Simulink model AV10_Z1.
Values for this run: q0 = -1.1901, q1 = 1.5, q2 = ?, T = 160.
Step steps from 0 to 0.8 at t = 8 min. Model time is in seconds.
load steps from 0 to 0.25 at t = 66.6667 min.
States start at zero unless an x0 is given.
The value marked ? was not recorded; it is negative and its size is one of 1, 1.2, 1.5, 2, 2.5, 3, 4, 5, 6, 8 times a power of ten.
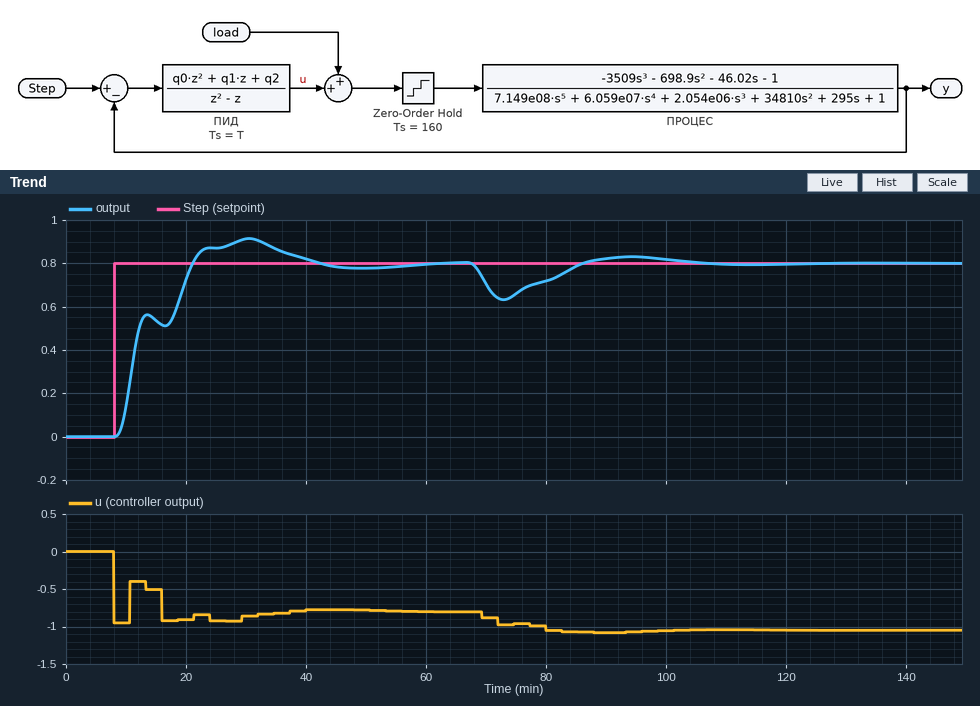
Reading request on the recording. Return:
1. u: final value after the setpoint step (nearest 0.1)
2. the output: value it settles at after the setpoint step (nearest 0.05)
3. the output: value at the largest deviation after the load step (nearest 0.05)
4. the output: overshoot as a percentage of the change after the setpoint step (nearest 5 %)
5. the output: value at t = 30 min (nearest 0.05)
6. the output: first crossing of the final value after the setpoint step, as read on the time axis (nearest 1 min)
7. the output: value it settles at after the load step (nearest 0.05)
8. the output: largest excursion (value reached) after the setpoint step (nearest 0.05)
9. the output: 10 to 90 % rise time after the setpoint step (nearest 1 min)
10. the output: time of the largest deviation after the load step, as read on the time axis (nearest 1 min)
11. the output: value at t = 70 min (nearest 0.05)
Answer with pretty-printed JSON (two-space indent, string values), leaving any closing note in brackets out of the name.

{
  "u: final value after the setpoint step": "-0.8",
  "the output: value it settles at after the setpoint step": "0.80",
  "the output: value at the largest deviation after the load step": "0.65",
  "the output: overshoot as a percentage of the change after the setpoint step": "15 %",
  "the output: value at t = 30 min": "0.90",
  "the output: first crossing of the final value after the setpoint step, as read on the time axis": "21 min",
  "the output: value it settles at after the load step": "0.80",
  "the output: largest excursion (value reached) after the setpoint step": "0.90",
  "the output: 10 to 90 % rise time after the setpoint step": "10 min",
  "the output: time of the largest deviation after the load step, as read on the time axis": "73 min",
  "the output: value at t = 70 min": "0.70"
}
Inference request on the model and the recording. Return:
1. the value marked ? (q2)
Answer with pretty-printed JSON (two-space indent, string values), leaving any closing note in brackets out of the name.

{
  "the value marked ?": "-0.8"
}
